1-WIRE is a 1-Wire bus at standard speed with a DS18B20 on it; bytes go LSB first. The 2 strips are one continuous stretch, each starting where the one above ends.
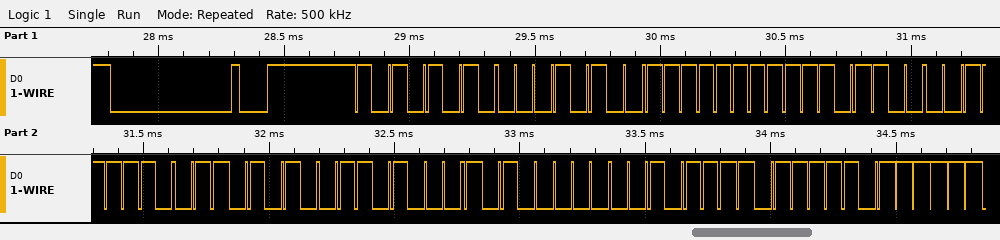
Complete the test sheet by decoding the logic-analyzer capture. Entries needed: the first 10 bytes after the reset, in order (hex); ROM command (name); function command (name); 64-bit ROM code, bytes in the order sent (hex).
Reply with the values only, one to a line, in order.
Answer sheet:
55 28 FF 37 7C 56 16 05 F4 BE
Match ROM
Read Scratchpad
28 FF 37 7C 56 16 05 F4
